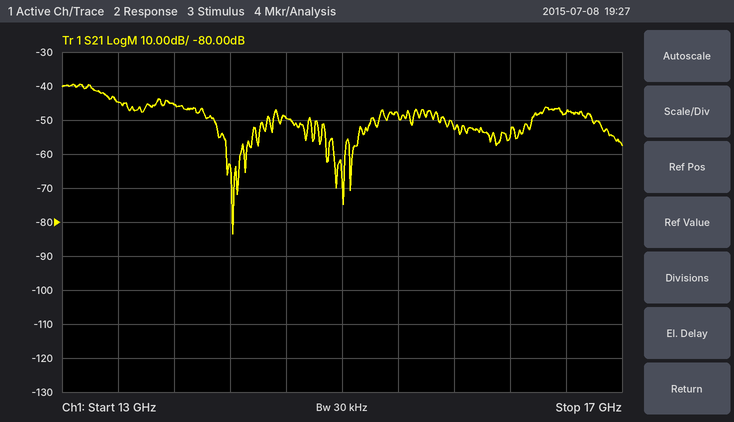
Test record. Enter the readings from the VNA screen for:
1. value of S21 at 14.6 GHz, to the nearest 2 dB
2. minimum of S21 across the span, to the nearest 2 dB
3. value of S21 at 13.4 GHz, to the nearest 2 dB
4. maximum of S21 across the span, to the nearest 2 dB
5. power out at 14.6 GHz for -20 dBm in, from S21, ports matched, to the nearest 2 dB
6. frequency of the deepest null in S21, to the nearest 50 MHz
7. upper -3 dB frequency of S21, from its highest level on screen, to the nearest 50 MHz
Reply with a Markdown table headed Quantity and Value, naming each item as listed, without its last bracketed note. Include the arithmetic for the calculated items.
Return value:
| Quantity | Value |
|---|---|
| value of S21 at 14.6 GHz, to the nearest 2 dB | -50 dB |
| minimum of S21 across the span, to the nearest 2 dB | -84 dB |
| value of S21 at 13.4 GHz, to the nearest 2 dB | -44 dB |
| maximum of S21 across the span, to the nearest 2 dB | -40 dB |
| power out at 14.6 GHz for -20 dBm in, from S21, ports matched, to the nearest 2 dB | -20 dBm + (-50 dB) = -70 dBm |
| frequency of the deepest null in S21, to the nearest 50 MHz | 14.20 GHz |
| upper -3 dB frequency of S21, from its highest level on screen, to the nearest 50 MHz | 13.30 GHz |
